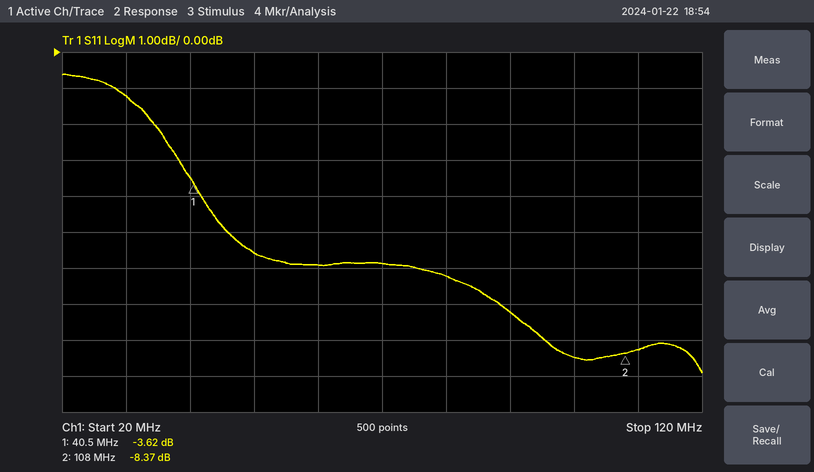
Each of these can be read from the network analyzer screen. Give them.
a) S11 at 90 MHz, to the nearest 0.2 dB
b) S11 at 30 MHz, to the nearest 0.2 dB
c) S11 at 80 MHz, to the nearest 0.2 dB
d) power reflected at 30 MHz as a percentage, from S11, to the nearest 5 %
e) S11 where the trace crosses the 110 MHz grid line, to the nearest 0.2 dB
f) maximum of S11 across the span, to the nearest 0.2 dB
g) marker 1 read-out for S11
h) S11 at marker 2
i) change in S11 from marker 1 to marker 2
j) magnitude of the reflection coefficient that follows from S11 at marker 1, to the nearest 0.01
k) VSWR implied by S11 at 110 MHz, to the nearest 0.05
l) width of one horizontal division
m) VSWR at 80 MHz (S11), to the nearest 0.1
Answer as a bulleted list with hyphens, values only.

- -7.2 dB
- -1.2 dB
- -6.2 dB
- 75 %
- -8.2 dB
- -0.6 dB
- -3.62 dB
- -8.37 dB
- -4.75 dB
- 0.66
- 2.25
- 10 MHz
- 2.9
